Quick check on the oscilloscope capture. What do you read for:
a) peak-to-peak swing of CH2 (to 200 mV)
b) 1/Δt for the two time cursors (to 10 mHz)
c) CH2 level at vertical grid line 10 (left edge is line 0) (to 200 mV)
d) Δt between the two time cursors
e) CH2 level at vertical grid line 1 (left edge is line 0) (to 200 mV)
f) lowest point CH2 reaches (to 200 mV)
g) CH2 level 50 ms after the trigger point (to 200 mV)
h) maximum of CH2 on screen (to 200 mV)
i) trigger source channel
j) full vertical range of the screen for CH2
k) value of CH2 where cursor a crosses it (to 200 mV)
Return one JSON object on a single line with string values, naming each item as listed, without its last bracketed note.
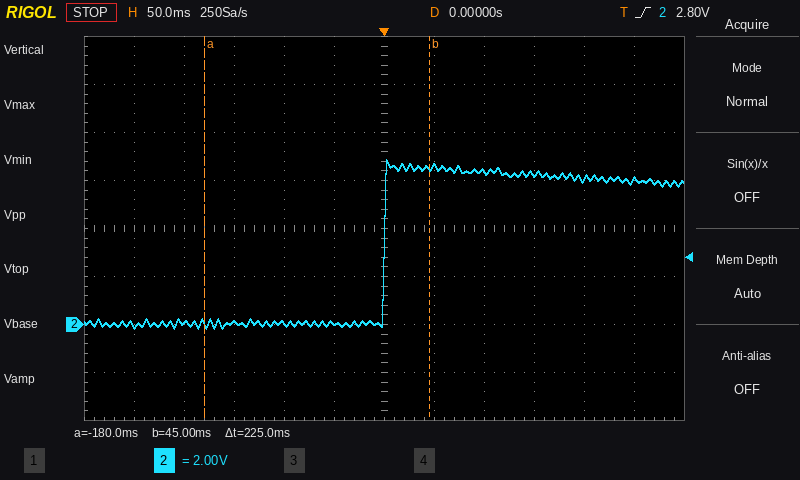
{"peak-to-peak swing of CH2": "7.0 V", "1/Δt for the two time cursors": "4.44 Hz", "CH2 level at vertical grid line 10 (left edge is line 0)": "6.0 V", "Δt between the two time cursors": "225 ms", "CH2 level at vertical grid line 1 (left edge is line 0)": "0.0 V", "lowest point CH2 reaches": "-200 mV", "CH2 level 50 ms after the trigger point": "6.6 V", "maximum of CH2 on screen": "6.8 V", "trigger source channel": "CH2", "full vertical range of the screen for CH2": "16 V", "value of CH2 where cursor a crosses it": "0.0 V"}
